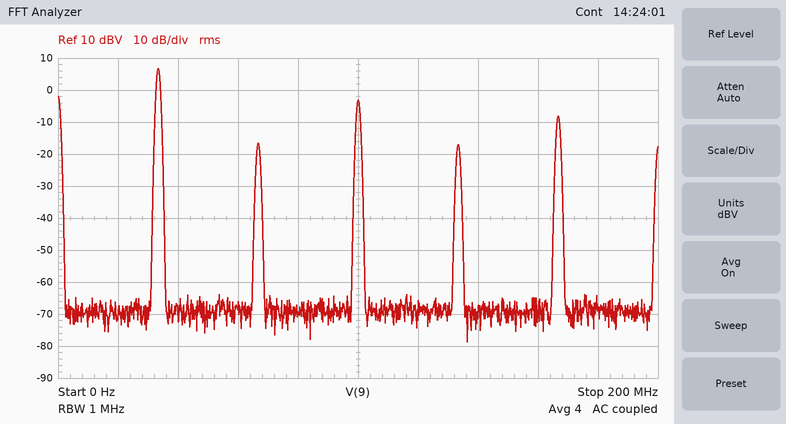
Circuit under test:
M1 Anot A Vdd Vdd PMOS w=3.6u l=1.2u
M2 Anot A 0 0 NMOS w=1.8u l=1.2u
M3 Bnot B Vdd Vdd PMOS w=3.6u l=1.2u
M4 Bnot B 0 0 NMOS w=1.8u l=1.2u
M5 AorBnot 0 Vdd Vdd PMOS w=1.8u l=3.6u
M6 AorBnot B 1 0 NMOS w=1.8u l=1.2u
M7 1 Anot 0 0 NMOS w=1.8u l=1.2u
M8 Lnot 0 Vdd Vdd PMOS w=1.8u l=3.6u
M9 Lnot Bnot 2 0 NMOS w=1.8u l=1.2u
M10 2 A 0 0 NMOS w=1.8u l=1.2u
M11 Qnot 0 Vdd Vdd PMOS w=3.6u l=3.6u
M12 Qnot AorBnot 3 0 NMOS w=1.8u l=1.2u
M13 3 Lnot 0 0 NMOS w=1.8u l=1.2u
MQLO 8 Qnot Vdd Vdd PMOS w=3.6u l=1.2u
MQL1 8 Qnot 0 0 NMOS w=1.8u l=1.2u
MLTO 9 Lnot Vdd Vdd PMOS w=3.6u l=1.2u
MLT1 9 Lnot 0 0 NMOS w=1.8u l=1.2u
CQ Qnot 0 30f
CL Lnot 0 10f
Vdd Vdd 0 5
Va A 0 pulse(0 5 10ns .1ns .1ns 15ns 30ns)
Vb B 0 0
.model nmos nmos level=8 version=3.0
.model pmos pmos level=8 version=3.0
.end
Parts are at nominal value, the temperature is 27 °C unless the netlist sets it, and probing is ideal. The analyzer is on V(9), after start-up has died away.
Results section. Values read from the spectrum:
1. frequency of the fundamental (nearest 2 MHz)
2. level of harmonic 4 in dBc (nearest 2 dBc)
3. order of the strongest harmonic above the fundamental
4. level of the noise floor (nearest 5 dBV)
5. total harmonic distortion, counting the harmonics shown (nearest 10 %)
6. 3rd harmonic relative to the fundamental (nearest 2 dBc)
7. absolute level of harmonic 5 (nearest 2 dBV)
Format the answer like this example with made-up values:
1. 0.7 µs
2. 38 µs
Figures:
1. 34 MHz
2. -24 dBc
3. 3
4. -70 dBV
5. 40 %
6. -10 dBc
7. -8 dBV
